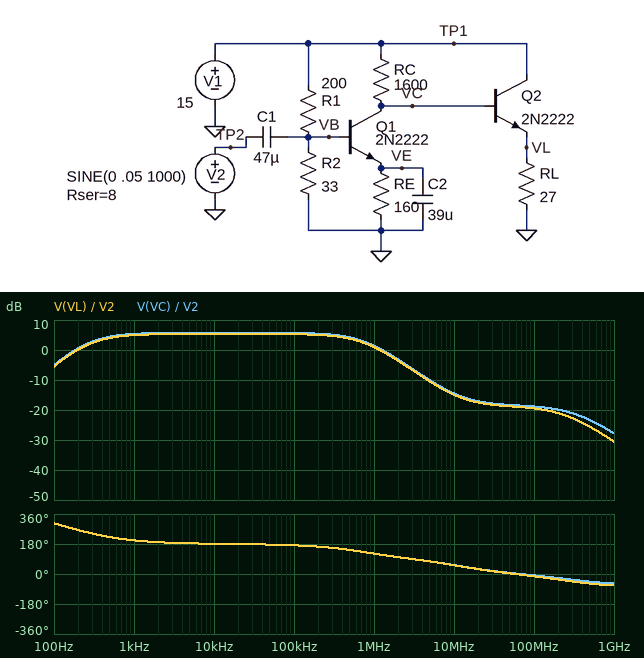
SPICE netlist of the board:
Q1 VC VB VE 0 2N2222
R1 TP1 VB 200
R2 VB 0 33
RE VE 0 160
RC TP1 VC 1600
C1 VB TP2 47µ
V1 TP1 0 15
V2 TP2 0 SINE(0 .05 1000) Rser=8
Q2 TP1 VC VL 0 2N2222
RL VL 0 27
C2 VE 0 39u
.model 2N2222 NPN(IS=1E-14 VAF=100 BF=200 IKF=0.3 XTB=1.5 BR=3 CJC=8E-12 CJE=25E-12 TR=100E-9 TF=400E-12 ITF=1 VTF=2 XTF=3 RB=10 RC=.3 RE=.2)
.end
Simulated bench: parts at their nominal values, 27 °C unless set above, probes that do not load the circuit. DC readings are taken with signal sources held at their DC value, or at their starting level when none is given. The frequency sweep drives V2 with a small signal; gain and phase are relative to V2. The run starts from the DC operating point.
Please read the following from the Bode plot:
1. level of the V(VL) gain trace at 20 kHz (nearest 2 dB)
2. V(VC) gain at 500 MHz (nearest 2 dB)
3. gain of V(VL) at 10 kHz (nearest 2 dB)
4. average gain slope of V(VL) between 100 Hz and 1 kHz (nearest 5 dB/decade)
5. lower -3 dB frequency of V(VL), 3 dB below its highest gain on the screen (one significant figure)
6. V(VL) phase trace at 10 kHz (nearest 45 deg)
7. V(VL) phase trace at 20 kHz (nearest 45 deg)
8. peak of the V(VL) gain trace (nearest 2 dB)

6 dB
-24 dB
6 dB
10 dB/decade
300 Hz
180 deg
180 deg
6 dB
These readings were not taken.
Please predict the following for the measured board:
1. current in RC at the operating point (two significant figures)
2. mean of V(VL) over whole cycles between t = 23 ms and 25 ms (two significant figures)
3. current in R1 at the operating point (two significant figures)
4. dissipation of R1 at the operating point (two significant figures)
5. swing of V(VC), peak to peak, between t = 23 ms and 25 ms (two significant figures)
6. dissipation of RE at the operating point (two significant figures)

8.5 mA
1.5 V
64 mA
830 mW
3.9 V
12 mW
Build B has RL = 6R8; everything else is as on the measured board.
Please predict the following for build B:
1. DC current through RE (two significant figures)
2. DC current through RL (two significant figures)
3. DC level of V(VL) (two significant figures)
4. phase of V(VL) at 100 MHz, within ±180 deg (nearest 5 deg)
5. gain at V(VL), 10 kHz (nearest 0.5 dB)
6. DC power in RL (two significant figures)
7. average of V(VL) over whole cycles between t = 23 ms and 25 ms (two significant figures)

8.6 mA
93 mA
630 mV
-30 deg
-1.5 dB
59 mW
870 mV
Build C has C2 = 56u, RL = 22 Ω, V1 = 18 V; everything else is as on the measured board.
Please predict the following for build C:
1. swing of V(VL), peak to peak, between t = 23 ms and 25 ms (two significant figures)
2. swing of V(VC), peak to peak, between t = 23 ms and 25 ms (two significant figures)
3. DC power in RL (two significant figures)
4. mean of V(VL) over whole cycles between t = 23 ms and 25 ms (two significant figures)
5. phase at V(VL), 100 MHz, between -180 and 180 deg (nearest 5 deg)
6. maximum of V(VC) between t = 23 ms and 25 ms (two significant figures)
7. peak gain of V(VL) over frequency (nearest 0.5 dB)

1.8 V
1.9 V
50 mW
1.3 V
-20 deg
3.7 V
-6.5 dB
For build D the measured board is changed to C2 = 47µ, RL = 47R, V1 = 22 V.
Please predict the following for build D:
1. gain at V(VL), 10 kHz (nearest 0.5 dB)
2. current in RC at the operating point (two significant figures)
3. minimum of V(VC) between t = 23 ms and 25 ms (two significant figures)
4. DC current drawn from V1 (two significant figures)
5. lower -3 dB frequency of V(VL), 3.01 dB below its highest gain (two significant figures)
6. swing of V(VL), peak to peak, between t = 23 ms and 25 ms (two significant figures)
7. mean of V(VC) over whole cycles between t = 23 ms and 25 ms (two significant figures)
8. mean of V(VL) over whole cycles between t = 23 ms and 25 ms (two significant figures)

-12.0 dB
12 mA
2.3 V
140 mA
50 Hz
39 mV
2.3 V
1.6 V
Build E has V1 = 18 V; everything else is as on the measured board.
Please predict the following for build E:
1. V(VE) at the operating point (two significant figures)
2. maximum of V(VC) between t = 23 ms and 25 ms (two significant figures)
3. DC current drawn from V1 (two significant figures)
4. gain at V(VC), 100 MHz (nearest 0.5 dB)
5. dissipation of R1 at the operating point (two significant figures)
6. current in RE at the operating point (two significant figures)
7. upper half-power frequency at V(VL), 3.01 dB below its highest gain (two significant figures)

1.8 V
3.8 V
130 mA
-21.5 dB
1.2 W
11 mA
710 kHz
